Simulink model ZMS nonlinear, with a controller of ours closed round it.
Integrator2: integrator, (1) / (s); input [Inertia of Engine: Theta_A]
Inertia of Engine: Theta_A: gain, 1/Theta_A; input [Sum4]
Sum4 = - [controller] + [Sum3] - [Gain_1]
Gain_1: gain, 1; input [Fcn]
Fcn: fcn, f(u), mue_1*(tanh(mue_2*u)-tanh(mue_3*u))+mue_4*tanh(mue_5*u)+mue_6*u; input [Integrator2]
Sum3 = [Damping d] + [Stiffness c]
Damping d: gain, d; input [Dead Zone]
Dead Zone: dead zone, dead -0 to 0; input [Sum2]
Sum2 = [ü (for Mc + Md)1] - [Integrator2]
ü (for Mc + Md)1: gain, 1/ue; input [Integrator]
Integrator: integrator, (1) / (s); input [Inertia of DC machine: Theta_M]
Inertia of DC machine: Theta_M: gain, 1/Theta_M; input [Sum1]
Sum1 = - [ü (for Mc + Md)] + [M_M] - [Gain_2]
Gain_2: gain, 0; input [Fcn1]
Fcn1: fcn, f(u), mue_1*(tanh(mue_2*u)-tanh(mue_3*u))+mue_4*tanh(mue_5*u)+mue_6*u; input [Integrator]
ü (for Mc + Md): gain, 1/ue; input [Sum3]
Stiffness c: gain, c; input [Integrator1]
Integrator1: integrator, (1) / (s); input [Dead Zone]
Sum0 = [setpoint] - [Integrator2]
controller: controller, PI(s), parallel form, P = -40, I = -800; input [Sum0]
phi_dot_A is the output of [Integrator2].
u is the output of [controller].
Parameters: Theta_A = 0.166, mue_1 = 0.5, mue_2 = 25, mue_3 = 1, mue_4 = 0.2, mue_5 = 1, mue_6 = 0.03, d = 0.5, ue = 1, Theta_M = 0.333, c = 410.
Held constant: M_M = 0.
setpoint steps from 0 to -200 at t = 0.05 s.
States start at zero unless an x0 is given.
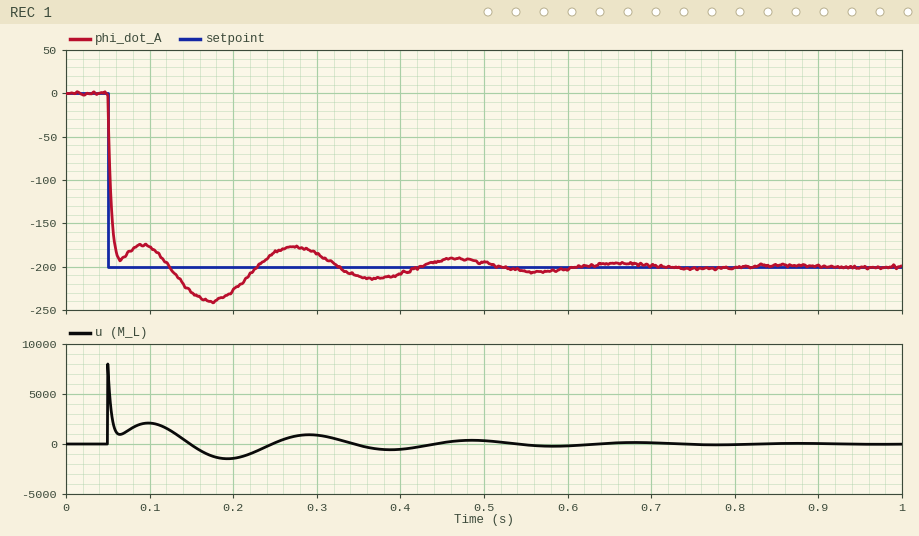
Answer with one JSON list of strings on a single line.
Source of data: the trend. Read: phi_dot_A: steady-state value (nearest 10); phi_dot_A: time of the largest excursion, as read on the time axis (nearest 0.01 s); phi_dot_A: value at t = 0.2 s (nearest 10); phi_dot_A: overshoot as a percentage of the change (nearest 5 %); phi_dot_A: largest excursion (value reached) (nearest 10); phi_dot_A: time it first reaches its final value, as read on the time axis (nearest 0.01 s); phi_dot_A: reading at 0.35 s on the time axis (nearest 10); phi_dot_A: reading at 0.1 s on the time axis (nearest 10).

["-200", "0.17 s", "-230", "20 %", "-240", "0.12 s", "-210", "-180"]
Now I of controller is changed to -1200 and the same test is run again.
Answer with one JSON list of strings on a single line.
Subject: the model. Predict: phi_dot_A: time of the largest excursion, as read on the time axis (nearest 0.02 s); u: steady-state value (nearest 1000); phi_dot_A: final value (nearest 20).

["0.16 s", "0", "-200"]
